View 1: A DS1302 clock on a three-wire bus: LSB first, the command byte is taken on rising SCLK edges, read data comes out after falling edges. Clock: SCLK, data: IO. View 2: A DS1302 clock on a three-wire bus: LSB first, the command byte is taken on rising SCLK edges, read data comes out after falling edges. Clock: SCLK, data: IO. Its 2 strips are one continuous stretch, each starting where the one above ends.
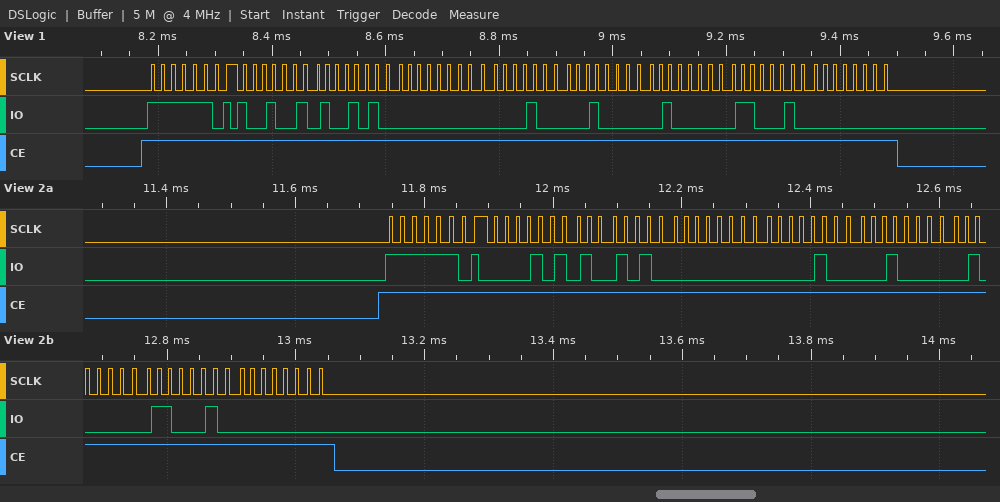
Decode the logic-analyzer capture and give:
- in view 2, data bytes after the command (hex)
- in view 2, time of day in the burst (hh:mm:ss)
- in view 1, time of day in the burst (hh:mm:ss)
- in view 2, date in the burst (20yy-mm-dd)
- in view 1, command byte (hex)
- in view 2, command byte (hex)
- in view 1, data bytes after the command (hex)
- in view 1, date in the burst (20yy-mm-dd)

50 29 00 10 04 02 23 00
00:29:50
00:29:49
2023-04-10
0xBF
0xBF
49 29 00 10 04 02 23 00
2023-04-10
